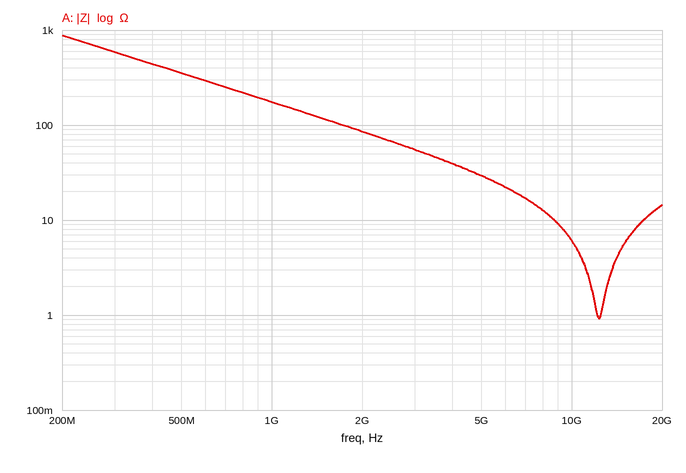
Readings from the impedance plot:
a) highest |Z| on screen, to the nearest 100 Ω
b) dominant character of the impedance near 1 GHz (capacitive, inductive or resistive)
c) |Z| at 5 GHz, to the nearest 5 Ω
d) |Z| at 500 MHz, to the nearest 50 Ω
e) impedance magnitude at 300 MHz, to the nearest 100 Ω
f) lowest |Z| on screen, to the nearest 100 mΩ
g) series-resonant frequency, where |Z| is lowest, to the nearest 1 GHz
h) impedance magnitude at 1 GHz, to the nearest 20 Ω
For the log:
900 Ω
capacitive
30 Ω
350 Ω
600 Ω
900 mΩ
12 GHz
180 Ω
